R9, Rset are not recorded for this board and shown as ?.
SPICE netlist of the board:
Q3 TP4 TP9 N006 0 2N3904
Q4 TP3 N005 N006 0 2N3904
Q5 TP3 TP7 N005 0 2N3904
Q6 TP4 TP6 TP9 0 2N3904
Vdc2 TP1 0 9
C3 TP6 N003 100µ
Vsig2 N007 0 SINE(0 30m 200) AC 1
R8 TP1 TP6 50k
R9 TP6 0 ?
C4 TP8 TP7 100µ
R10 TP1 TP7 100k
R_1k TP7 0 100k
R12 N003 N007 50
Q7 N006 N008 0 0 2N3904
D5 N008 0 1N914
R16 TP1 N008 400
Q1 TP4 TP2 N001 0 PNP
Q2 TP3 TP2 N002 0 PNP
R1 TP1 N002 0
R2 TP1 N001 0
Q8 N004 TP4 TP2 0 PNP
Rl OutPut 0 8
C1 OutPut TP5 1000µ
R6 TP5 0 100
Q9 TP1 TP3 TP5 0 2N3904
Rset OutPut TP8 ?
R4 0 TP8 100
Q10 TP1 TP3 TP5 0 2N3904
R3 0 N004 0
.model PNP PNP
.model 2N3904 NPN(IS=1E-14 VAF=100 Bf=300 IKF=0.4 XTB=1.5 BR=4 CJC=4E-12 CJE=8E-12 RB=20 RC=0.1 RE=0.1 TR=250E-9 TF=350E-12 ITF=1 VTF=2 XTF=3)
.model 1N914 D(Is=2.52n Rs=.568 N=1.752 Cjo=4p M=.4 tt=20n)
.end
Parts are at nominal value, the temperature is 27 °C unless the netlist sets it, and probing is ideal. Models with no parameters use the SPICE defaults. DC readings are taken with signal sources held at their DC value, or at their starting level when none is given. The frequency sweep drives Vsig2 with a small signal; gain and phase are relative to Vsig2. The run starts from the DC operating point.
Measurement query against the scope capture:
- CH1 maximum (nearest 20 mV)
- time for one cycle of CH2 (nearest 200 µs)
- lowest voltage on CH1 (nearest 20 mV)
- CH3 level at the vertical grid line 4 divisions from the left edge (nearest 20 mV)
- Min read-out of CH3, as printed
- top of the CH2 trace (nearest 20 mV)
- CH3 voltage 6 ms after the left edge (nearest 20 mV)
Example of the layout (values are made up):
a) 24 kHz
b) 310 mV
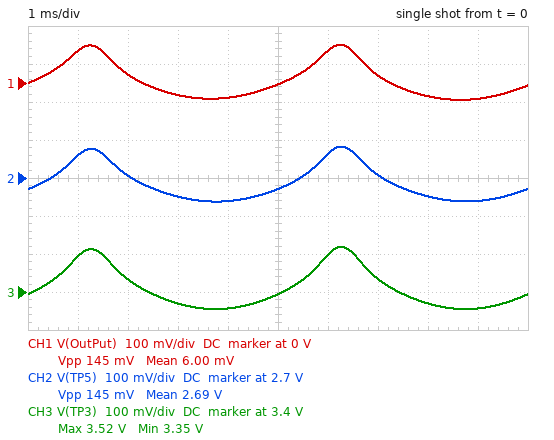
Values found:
a) 100 mV
b) 5.0 ms
c) -40 mV
d) 3.36 V
e) 3.35 V
f) 2.78 V
g) 3.50 V
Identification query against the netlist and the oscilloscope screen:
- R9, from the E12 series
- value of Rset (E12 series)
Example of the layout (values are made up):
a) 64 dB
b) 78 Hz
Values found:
a) 39 kΩ
b) 1.5 kΩ
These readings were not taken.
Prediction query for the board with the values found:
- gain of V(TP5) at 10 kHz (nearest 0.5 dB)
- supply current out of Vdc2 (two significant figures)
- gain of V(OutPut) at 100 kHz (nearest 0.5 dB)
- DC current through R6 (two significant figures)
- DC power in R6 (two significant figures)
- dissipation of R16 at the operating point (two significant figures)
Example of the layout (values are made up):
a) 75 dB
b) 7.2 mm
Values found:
a) 3.0 dB
b) 66 mA
c) 3.0 dB
d) 27 mA
e) 71 mW
f) 170 mW
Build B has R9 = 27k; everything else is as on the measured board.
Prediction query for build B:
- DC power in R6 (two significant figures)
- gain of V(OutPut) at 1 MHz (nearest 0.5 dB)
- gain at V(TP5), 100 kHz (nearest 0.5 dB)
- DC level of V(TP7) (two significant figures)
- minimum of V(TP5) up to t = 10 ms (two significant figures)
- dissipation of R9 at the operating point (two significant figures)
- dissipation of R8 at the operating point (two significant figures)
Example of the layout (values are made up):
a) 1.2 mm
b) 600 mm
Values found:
a) 36 mW
b) -0.5 dB
c) 0 dB
d) 3.2 V
e) 1.9 V
f) 370 µW
g) 680 µW
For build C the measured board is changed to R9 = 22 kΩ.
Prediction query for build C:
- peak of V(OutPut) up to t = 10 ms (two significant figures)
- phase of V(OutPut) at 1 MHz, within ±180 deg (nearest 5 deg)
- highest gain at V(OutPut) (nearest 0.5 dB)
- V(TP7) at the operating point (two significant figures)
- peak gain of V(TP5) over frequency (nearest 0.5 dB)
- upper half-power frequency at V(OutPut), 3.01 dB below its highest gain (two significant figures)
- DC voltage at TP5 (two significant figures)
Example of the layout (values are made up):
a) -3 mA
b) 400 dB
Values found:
a) 31 mV
b) -5 deg
c) -0.5 dB
d) 2.8 V
e) 1.0 dB
f) 20 MHz
g) 1.5 V
